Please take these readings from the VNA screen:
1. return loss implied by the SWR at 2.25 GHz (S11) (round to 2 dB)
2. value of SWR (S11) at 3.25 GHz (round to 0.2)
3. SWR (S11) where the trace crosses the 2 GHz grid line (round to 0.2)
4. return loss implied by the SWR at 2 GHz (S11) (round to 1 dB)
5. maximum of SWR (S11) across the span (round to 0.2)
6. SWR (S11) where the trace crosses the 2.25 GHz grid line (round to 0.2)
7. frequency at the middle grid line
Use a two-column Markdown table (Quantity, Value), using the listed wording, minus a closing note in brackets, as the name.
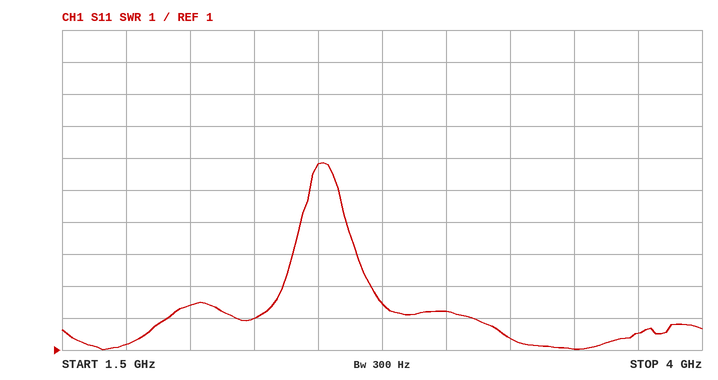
| Quantity | Value |
|---|---|
| return loss implied by the SWR at 2.25 GHz (S11) | 10 dB |
| value of SWR (S11) at 3.25 GHz | 1.4 |
| SWR (S11) where the trace crosses the 2 GHz grid line | 2.4 |
| return loss implied by the SWR at 2 GHz (S11) | 8 dB |
| maximum of SWR (S11) across the span | 6.8 |
| SWR (S11) where the trace crosses the 2.25 GHz grid line | 2.0 |
| frequency at the middle grid line | 2.75 GHz |
